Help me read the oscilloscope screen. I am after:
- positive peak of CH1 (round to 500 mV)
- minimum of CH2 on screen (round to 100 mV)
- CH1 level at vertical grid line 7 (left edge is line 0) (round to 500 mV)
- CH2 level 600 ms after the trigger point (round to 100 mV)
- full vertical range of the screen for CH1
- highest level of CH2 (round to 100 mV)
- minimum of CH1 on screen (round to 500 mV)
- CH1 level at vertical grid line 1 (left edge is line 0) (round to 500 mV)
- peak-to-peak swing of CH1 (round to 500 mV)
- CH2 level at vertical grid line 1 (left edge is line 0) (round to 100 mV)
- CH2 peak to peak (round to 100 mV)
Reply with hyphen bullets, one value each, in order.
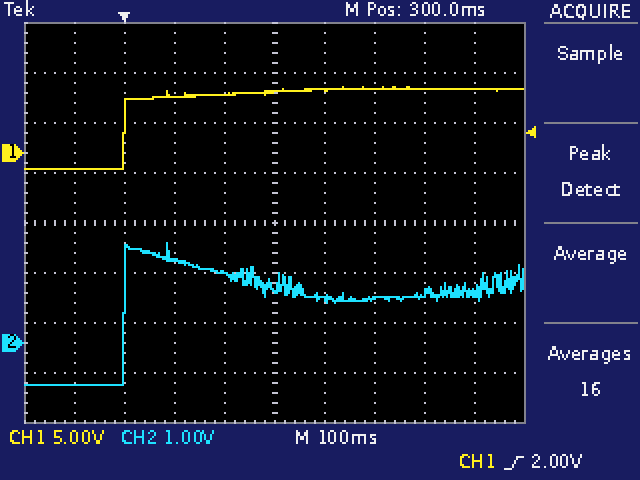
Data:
- 6.5 V
- -800 mV
- 6.5 V
- 1.0 V
- 40 V
- 2.0 V
- -1.5 V
- -1.5 V
- 8.0 V
- -800 mV
- 2.8 V
